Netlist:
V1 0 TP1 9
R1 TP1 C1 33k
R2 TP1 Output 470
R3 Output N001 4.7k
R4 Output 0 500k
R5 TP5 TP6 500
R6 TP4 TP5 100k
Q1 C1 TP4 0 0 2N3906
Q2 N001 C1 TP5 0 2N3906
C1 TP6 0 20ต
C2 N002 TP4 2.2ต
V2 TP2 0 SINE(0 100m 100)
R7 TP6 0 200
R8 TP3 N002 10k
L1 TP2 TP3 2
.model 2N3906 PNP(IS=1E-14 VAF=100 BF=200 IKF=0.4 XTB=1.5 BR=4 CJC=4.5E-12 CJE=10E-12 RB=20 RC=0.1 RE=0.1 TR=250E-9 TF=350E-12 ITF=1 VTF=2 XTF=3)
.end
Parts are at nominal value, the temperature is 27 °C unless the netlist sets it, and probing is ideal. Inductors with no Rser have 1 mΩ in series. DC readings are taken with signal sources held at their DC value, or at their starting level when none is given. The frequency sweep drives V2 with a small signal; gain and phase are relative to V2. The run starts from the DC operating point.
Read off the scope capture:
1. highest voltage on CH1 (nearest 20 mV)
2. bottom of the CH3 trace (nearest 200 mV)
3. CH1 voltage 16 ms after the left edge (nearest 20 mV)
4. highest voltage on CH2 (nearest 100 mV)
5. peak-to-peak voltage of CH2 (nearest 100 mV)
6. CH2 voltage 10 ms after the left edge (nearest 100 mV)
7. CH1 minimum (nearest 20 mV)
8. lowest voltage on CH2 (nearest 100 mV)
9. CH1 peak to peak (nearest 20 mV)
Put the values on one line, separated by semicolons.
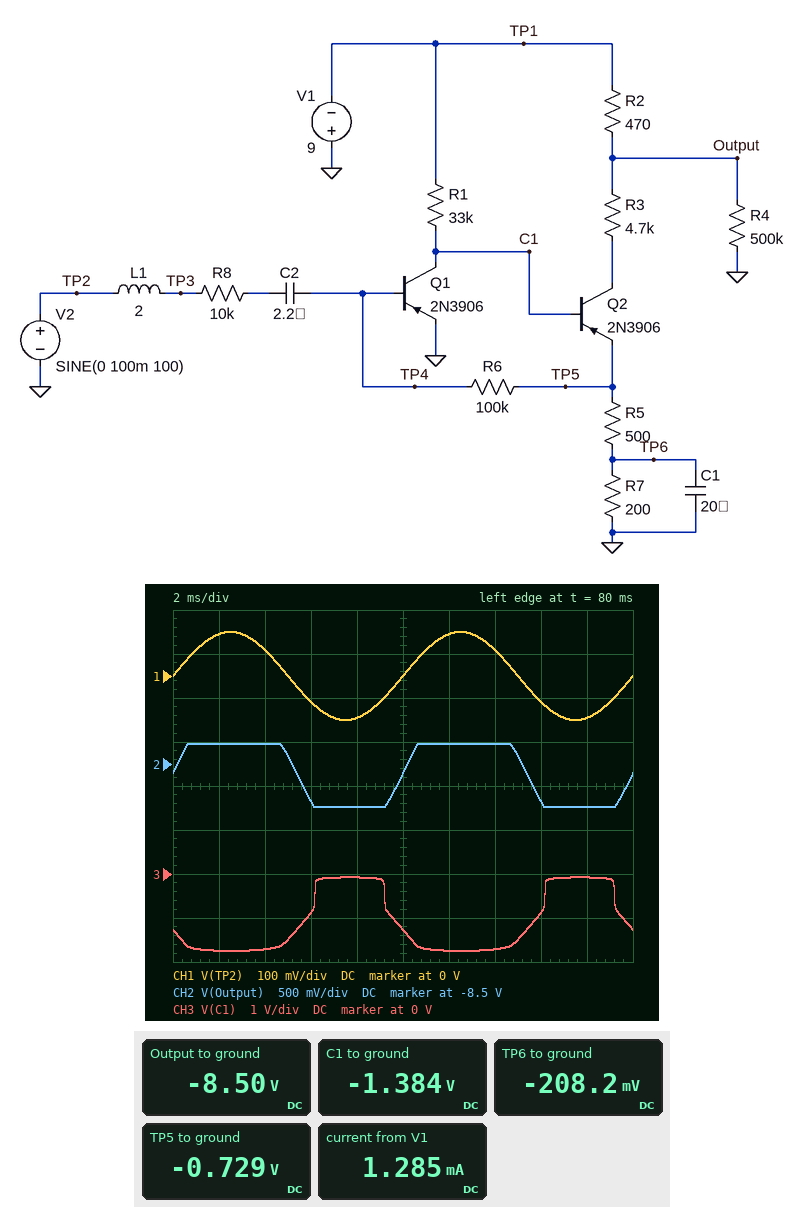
100 mV; -1.8 V; -60 mV; -8.3 V; 700 mV; -8.6 V; -100 mV; -9.0 V; 200 mV
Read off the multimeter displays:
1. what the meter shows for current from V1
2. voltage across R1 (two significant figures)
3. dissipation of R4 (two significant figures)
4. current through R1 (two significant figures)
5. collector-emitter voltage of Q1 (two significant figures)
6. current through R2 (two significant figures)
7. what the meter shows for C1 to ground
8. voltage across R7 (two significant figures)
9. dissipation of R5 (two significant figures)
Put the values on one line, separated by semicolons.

1.285 mA; 7.6 V; 140 µW; 230 µA; -1.4 V; 1.1 mA; -1.384 V; 210 mV; 540 µW
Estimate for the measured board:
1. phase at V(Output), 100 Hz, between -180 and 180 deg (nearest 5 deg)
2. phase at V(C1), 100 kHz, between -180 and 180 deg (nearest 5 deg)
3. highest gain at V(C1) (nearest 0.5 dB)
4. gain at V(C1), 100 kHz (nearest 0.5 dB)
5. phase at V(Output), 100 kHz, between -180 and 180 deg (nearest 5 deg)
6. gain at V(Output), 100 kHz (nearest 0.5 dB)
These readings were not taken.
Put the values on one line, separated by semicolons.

-5 deg; 75 deg; 20.0 dB; -22.0 dB; -105 deg; -23.0 dB
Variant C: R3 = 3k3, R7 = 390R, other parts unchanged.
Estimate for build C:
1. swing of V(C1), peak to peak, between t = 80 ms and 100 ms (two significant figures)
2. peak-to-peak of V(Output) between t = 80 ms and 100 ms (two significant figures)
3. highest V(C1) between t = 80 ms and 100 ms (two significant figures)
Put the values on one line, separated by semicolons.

2.0 V; 940 mV; -71 mV
